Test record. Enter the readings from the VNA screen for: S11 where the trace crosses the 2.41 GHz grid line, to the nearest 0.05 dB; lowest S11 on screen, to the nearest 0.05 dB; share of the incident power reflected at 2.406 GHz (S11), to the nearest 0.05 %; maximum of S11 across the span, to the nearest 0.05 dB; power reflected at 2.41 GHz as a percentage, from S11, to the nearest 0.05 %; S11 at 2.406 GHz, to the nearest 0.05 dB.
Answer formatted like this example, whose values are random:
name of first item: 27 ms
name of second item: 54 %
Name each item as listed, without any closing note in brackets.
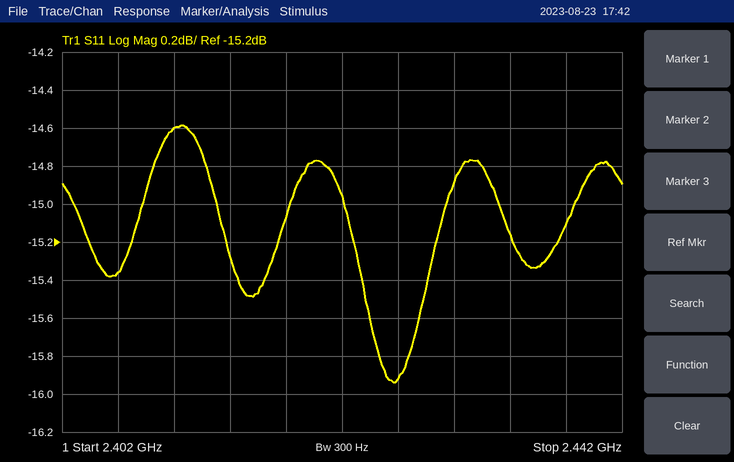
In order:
S11 where the trace crosses the 2.41 GHz grid line, to the nearest 0.05 dB: -14.60 dB
lowest S11 on screen, to the nearest 0.05 dB: -15.95 dB
share of the incident power reflected at 2.406 GHz (S11), to the nearest 0.05 %: 2.90 %
maximum of S11 across the span, to the nearest 0.05 dB: -14.60 dB
power reflected at 2.41 GHz as a percentage, from S11, to the nearest 0.05 %: 3.45 %
S11 at 2.406 GHz, to the nearest 0.05 dB: -15.35 dB
